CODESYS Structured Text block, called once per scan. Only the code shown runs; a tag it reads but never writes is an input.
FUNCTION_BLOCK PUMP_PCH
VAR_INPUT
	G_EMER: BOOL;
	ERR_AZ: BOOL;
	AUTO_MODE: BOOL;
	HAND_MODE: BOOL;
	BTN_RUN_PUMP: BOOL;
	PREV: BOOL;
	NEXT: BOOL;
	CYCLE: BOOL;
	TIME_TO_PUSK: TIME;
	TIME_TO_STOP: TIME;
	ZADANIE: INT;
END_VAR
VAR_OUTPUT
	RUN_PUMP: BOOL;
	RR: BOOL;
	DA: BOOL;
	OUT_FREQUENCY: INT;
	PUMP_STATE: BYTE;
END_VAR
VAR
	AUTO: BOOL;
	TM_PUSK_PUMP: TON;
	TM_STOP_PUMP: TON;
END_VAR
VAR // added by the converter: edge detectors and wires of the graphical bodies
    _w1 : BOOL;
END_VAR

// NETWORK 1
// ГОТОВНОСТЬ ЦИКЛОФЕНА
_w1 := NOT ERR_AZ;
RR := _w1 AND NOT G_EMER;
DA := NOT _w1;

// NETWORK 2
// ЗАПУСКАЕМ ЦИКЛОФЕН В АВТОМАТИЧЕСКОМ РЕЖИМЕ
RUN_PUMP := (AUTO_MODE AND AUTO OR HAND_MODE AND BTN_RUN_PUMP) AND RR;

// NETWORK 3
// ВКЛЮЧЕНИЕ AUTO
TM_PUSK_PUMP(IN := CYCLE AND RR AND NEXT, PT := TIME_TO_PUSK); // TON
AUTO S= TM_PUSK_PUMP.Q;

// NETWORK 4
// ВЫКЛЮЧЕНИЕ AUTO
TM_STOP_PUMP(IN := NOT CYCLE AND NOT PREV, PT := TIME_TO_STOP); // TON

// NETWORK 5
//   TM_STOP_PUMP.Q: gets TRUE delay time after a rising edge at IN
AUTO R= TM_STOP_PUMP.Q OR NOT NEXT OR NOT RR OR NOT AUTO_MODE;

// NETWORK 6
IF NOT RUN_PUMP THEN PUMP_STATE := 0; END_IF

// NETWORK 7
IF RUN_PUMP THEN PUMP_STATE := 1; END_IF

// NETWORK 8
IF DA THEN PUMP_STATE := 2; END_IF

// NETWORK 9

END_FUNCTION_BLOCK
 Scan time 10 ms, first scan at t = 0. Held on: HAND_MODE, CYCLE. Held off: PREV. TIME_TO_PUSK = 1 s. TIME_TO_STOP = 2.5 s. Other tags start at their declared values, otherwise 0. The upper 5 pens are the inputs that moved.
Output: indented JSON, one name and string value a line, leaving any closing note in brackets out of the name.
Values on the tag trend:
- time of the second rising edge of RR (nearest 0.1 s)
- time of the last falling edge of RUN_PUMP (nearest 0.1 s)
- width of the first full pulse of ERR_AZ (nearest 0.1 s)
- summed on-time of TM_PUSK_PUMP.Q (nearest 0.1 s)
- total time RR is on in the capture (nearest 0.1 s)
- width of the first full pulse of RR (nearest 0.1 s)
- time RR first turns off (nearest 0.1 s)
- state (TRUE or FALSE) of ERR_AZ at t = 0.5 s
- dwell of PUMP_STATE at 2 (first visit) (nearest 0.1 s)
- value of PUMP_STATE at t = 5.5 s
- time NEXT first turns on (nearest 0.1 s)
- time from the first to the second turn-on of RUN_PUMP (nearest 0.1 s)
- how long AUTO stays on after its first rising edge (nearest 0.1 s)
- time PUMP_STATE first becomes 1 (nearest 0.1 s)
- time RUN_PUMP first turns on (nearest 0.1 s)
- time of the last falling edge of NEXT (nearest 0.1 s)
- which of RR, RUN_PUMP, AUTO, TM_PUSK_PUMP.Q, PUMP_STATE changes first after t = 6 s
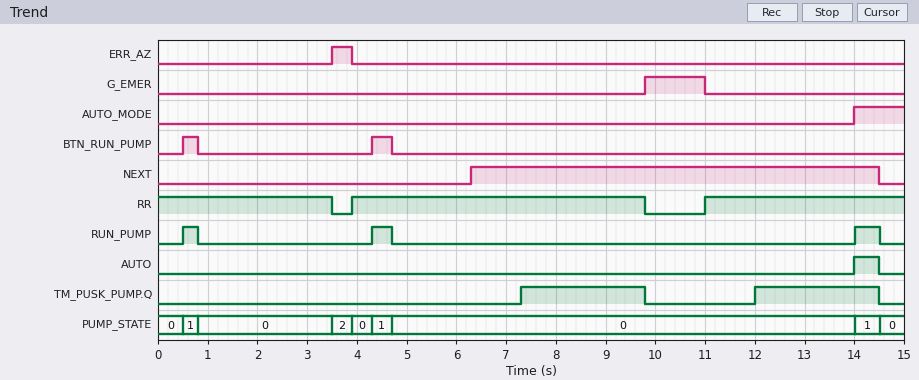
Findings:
{
  "time of the second rising edge of RR": "11.0 s",
  "time of the last falling edge of RUN_PUMP": "14.5 s",
  "width of the first full pulse of ERR_AZ": "0.4 s",
  "summed on-time of TM_PUSK_PUMP.Q": "5.0 s",
  "total time RR is on in the capture": "13.4 s",
  "width of the first full pulse of RR": "5.9 s",
  "time RR first turns off": "3.5 s",
  "state (TRUE or FALSE) of ERR_AZ at t = 0.5 s": "FALSE",
  "dwell of PUMP_STATE at 2 (first visit)": "0.4 s",
  "value of PUMP_STATE at t = 5.5 s": "0",
  "time NEXT first turns on": "6.3 s",
  "time from the first to the second turn-on of RUN_PUMP": "3.8 s",
  "how long AUTO stays on after its first rising edge": "0.5 s",
  "time PUMP_STATE first becomes 1": "0.5 s",
  "time RUN_PUMP first turns on": "0.5 s",
  "time of the last falling edge of NEXT": "14.5 s",
  "which of RR, RUN_PUMP, AUTO, TM_PUSK_PUMP.Q, PUMP_STATE changes first after t = 6 s": "TM_PUSK_PUMP.Q"
}
